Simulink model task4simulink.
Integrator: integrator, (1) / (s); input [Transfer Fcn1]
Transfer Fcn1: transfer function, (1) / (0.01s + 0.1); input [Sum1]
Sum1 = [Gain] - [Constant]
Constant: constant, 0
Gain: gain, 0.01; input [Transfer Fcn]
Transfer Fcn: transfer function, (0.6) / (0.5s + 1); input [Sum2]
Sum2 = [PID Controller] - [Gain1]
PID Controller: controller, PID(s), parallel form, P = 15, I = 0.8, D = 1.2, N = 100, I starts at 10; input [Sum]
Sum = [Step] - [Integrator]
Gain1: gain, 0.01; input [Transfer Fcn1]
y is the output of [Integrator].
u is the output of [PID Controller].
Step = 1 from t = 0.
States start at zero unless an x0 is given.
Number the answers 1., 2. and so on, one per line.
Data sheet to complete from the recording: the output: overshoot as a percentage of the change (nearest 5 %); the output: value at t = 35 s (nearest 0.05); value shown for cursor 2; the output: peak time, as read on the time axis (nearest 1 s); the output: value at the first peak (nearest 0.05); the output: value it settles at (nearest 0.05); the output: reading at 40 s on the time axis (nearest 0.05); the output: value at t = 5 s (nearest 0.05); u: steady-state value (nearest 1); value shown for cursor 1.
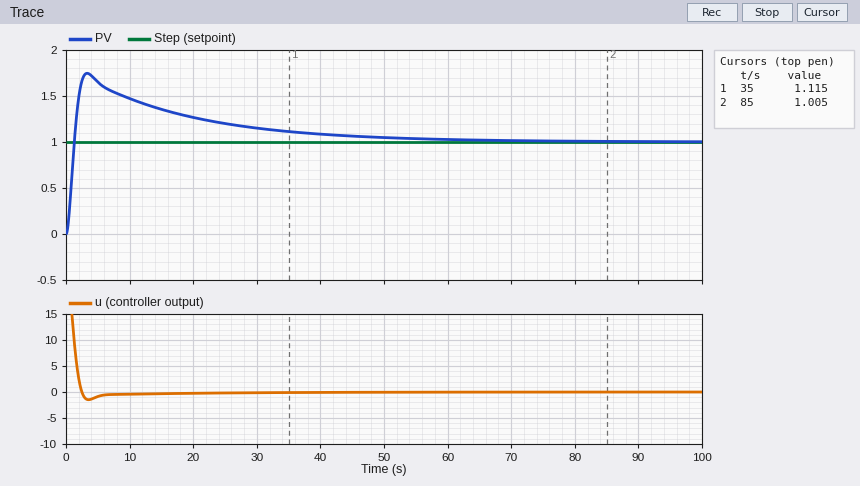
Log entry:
1. 75 %
2. 1.10
3. 1.005
4. 3 s
5. 1.75
6. 1.00
7. 1.10
8. 1.65
9. 0
10. 1.115
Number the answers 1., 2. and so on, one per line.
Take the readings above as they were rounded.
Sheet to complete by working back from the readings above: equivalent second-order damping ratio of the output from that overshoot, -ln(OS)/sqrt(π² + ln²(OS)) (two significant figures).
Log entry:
1. 0.091
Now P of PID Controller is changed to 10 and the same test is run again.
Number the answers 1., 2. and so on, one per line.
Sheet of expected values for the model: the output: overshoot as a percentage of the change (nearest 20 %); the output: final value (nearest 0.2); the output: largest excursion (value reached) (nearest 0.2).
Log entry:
1. 100 %
2. 1.0
3. 2.0
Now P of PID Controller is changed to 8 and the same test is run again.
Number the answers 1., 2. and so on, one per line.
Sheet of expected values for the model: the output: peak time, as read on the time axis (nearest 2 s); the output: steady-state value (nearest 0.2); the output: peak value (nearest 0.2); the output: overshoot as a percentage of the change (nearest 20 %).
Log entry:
1. 6 s
2. 1.0
3. 2.2
4. 120 %
